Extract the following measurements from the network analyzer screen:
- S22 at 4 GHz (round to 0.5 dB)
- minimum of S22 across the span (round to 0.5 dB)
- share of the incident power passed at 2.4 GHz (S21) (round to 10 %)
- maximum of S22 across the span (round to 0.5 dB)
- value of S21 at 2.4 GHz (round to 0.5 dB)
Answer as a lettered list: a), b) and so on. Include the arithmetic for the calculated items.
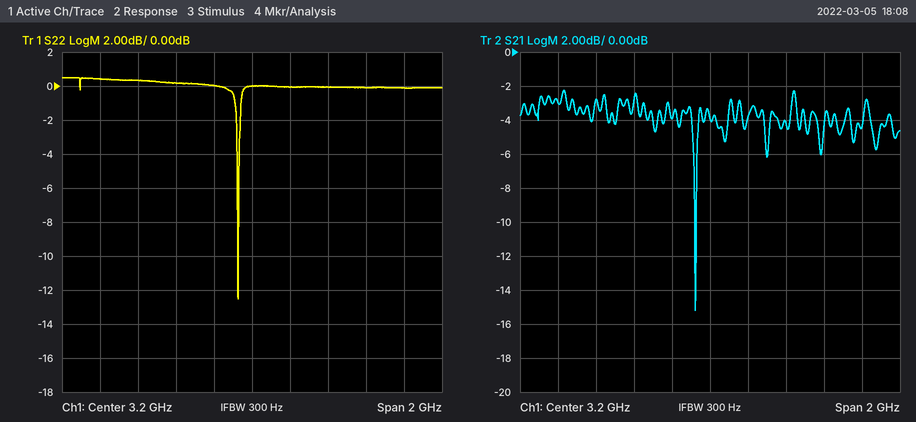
a) 0.0 dB
b) -12.5 dB
c) 10^(-3/10) ≈ 50 %
d) 0.5 dB
e) -3.0 dB
